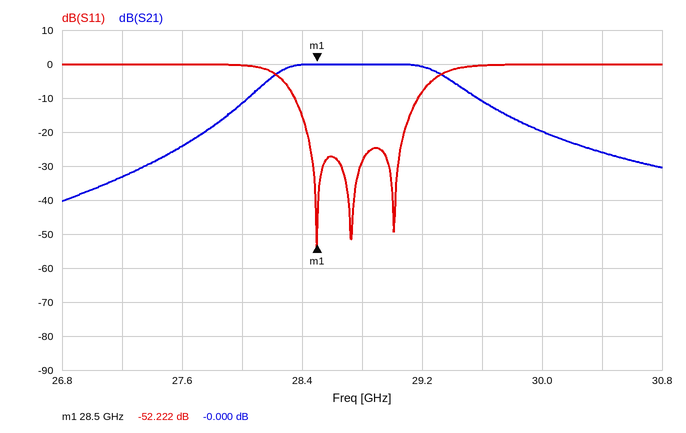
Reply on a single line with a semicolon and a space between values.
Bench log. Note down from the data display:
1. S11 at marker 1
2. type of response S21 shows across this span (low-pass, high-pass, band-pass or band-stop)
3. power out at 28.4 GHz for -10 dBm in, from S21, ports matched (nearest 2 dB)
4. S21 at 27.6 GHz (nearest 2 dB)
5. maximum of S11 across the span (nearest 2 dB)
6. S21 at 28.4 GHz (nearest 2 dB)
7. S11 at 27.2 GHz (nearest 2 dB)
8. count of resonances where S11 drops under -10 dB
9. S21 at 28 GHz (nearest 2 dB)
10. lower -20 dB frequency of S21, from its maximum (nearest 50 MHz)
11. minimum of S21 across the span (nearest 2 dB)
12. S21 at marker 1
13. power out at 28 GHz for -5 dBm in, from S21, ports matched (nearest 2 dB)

-52.222 dB; band-pass; -10 dBm; -24 dB; 0 dB; 0 dB; 0 dB; 3; -12 dB; 27.75 GHz; -40 dB; -0.000 dB; -16 dBm
